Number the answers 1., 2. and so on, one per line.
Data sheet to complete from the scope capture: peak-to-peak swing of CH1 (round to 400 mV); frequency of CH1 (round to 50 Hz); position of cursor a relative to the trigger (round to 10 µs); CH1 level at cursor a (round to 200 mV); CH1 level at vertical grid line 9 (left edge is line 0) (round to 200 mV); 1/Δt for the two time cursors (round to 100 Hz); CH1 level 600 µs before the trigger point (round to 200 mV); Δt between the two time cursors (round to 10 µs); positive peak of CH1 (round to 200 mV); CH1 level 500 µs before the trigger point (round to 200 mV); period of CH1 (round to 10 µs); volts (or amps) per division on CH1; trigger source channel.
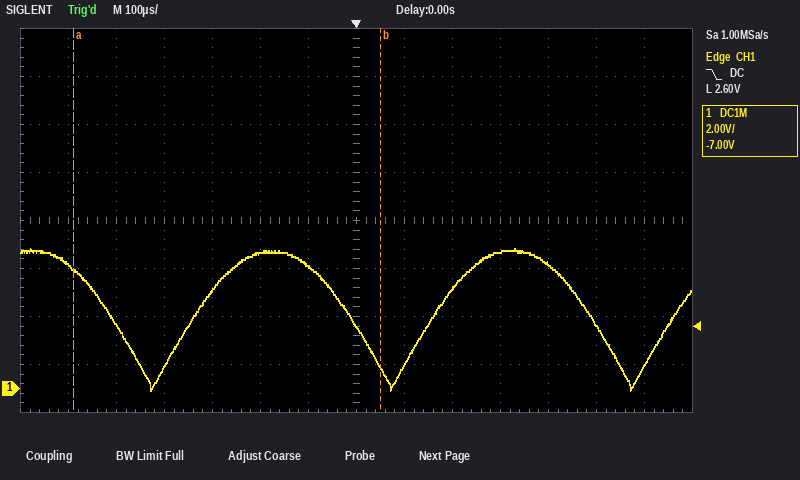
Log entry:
1. 6.0 V
2. 2.00 kHz
3. -590 µs
4. 5.0 V
5. 4.2 V
6. 1.6 kHz
7. 5.2 V
8. 640 µs
9. 5.8 V
10. 2.6 V
11. 500 µs
12. 2 V
13. CH1
